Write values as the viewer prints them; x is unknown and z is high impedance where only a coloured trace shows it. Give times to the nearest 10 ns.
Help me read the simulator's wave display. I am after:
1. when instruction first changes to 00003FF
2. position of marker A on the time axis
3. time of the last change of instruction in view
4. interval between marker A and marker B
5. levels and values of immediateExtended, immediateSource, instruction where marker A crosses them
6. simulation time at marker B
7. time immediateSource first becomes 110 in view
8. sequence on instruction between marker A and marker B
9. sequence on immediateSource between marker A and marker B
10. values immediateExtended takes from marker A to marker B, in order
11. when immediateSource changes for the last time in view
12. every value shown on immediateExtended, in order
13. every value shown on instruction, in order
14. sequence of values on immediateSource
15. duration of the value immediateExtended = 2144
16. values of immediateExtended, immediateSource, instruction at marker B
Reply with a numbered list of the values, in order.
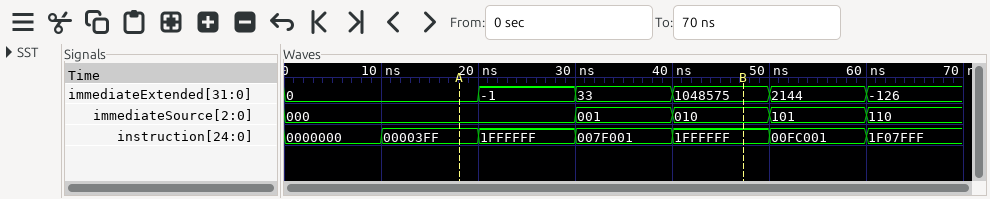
1. 10 ns
2. 20 ns
3. 60 ns
4. 30 ns
5. immediateExtended=0, immediateSource=000, instruction=00003FF
6. 50 ns
7. 60 ns
8. 00003FF, 1FFFFFF, 007F001, 1FFFFFF
9. 000, 001, 010
10. 0, -1, 33, 1048575
11. 60 ns
12. 0, -1, 33, 1048575, 2144, -126
13. 0000000, 00003FF, 1FFFFFF, 007F001, 1FFFFFF, 00FC001, 1F07FFF
14. 000, 001, 010, 101, 110
15. 10 ns
16. immediateExtended=1048575, immediateSource=010, instruction=1FFFFFF
